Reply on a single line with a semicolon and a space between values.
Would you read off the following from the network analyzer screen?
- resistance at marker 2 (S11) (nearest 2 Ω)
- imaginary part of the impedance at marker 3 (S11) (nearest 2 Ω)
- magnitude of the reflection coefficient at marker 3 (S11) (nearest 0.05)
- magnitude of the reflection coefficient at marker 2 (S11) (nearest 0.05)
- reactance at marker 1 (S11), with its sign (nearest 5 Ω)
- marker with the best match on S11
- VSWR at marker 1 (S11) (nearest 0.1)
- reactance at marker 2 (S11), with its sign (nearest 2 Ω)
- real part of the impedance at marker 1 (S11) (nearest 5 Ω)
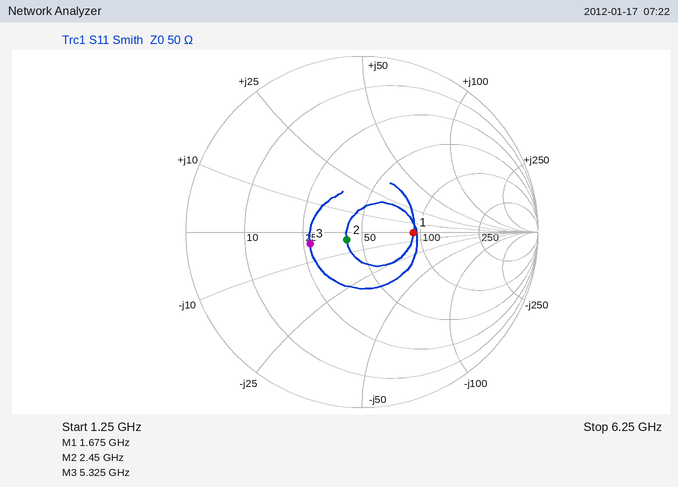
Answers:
42 Ω; -4 Ω; 0.30; 0.10; 0 Ω; marker 2; 1.8; -4 Ω; 90 Ω
